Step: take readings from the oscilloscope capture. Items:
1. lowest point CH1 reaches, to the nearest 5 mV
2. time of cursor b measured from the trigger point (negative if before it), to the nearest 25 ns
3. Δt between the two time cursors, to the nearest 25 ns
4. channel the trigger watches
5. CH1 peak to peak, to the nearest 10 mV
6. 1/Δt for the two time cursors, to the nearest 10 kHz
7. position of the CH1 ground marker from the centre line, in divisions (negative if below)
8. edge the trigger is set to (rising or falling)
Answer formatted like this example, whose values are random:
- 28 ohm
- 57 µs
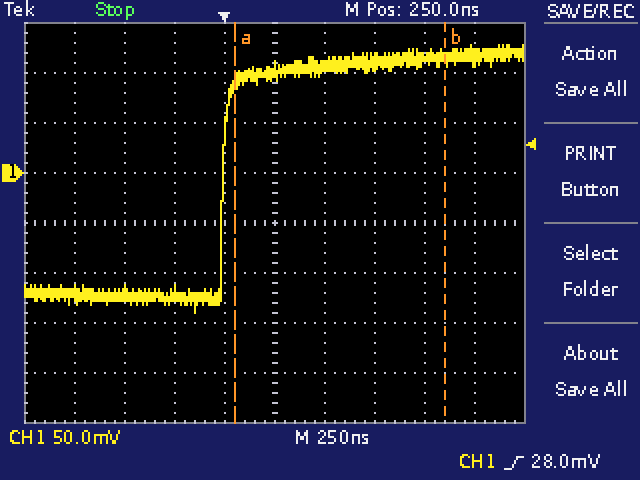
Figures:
- -140 mV
- +1.100 µs
- 1.050 µs
- CH1
- 270 mV
- 950 kHz
- +1.0 div
- rising
